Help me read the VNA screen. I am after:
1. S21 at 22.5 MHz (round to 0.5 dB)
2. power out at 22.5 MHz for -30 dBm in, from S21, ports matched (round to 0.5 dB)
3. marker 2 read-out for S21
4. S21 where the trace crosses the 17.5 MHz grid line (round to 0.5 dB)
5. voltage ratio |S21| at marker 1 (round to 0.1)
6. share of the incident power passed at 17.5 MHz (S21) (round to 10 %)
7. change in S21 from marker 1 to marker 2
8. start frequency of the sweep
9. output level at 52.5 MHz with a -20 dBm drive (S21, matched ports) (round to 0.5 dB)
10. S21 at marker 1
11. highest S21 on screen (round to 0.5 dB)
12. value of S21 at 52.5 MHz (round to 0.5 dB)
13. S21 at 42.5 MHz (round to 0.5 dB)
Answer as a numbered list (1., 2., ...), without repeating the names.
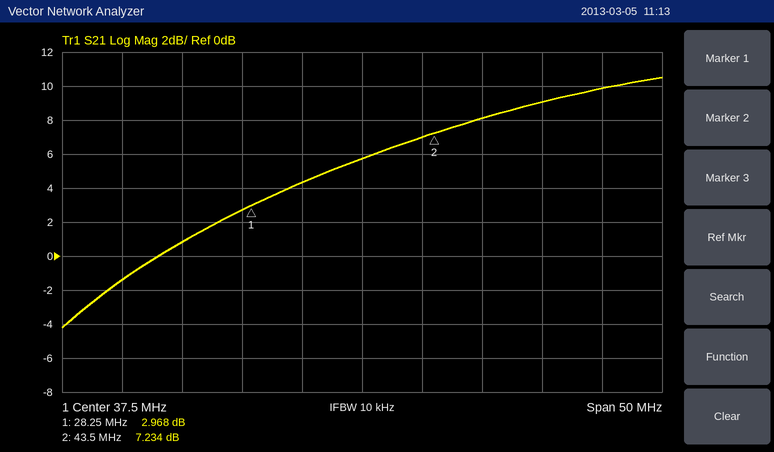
1. 1.0 dB
2. -29.0 dBm
3. 7.234 dB
4. -1.5 dB
5. 1.4
6. 70 %
7. 4.266 dB
8. 12.5 MHz
9. -11.0 dBm
10. 2.968 dB
11. 10.5 dB
12. 9.0 dB
13. 7.0 dB
